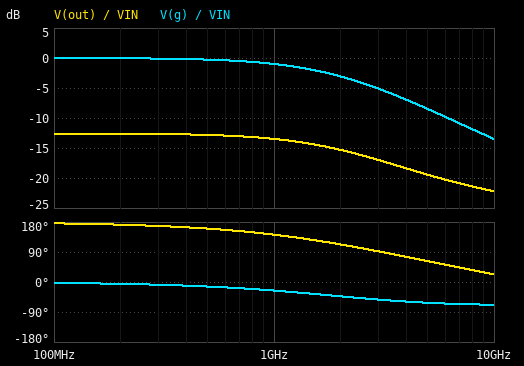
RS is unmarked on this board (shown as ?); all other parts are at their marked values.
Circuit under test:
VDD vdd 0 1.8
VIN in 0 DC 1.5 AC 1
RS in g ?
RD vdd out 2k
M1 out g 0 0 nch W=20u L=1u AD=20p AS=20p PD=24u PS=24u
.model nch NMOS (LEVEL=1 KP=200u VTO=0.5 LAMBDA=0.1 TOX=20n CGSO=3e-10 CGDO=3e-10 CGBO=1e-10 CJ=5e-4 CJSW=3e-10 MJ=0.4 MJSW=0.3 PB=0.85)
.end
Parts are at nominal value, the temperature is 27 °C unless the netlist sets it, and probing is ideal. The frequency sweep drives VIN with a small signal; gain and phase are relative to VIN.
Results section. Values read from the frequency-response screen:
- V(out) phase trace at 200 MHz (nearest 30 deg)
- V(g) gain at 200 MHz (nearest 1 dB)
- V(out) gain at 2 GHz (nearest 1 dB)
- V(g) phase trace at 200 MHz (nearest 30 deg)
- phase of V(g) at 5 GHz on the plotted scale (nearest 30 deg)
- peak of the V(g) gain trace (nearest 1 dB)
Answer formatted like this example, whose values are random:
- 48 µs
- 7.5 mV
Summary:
- 180 deg
- 0 dB
- -15 dB
- 0 deg
- -60 deg
- 0 dB
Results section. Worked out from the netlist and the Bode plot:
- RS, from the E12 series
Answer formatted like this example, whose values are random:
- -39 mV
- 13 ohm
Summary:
- 1.5 kΩ
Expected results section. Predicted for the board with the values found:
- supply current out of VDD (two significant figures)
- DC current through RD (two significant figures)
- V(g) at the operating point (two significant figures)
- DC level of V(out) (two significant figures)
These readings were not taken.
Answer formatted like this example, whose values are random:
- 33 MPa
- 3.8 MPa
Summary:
- 790 µA
- 790 µA
- 1.5 V
- 220 mV
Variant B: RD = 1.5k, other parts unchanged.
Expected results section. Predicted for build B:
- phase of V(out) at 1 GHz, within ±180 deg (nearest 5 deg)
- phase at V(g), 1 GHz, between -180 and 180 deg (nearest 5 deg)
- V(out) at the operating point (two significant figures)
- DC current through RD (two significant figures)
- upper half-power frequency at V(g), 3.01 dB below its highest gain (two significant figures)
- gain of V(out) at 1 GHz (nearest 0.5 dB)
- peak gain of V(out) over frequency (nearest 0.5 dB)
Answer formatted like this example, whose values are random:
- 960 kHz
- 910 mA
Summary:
- 145 deg
- -25 deg
- 290 mV
- 1.0 mA
- 1.9 GHz
- -11.0 dB
- -10.0 dB
